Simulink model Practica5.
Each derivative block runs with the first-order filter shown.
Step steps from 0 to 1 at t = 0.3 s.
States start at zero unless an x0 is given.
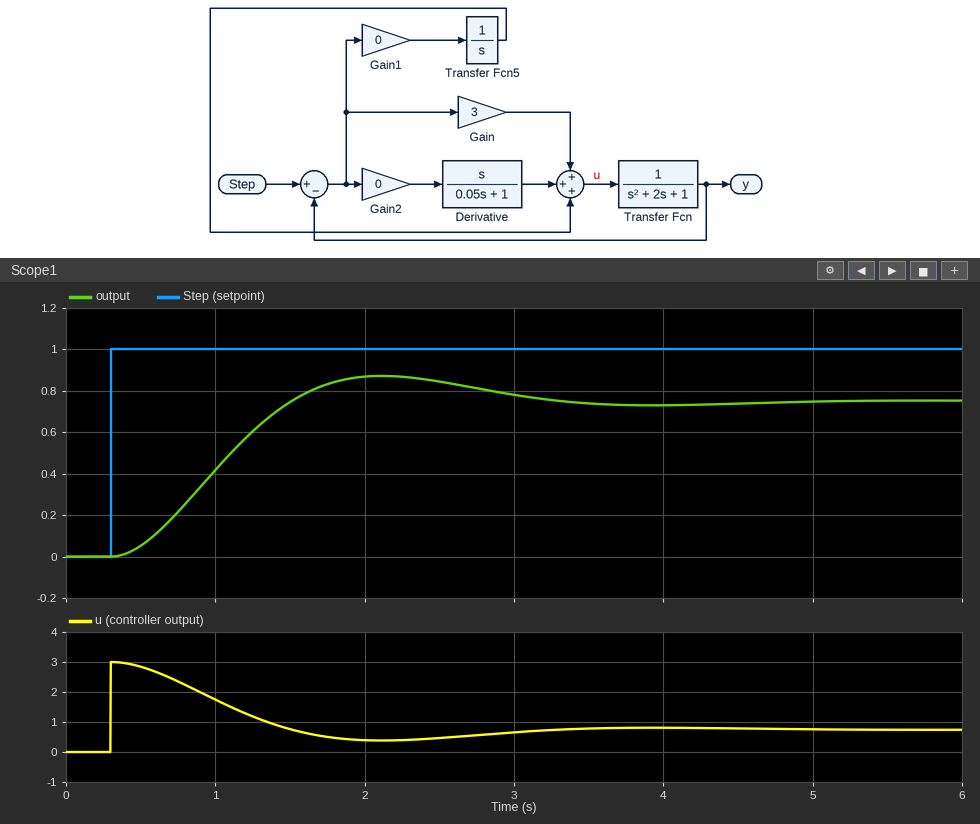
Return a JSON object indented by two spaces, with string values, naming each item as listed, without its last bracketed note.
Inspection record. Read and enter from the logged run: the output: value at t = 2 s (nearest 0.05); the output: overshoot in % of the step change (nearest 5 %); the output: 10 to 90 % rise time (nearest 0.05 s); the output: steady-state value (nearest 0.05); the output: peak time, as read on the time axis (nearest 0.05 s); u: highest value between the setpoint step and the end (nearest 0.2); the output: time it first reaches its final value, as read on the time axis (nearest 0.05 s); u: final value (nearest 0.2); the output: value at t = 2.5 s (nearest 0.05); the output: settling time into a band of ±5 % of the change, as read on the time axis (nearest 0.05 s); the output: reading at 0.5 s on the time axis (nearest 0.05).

{
  "the output: value at t = 2 s": "0.85",
  "the output: overshoot in % of the step change": "15 %",
  "the output: 10 to 90 % rise time": "0.80 s",
  "the output: steady-state value": "0.75",
  "the output: peak time, as read on the time axis": "2.10 s",
  "u: highest value between the setpoint step and the end": "3.0",
  "the output: time it first reaches its final value, as read on the time axis": "1.50 s",
  "u: final value": "0.8",
  "the output: value at t = 2.5 s": "0.85",
  "the output: settling time into a band of ±5 % of the change, as read on the time axis": "2.95 s",
  "the output: reading at 0.5 s on the time axis": "0.05"
}
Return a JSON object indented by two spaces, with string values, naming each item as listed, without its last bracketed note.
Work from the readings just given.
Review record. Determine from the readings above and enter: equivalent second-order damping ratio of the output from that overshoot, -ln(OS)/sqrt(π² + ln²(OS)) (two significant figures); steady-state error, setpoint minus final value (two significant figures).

{
  "equivalent second-order damping ratio of the output from that overshoot, -ln(OS)/sqrt(π² + ln²(OS))": "0.52",
  "steady-state error, setpoint minus final value": "0.25"
}
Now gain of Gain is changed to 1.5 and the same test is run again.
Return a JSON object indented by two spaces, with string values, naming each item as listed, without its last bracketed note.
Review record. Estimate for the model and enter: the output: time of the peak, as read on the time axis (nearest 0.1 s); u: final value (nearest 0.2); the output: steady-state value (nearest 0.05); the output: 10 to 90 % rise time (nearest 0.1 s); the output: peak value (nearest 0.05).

{
  "the output: time of the peak, as read on the time axis": "2.9 s",
  "u: final value": "0.6",
  "the output: steady-state value": "0.60",
  "the output: 10 to 90 % rise time": "1.2 s",
  "the output: peak value": "0.65"
}
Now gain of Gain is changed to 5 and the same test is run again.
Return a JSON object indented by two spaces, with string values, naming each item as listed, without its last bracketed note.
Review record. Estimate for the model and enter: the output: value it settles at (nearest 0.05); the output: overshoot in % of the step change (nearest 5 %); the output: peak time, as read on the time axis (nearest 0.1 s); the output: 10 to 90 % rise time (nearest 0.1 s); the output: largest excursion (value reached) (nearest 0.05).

{
  "the output: value it settles at": "0.85",
  "the output: overshoot in % of the step change": "25 %",
  "the output: peak time, as read on the time axis": "1.7 s",
  "the output: 10 to 90 % rise time": "0.6 s",
  "the output: largest excursion (value reached)": "1.05"
}
